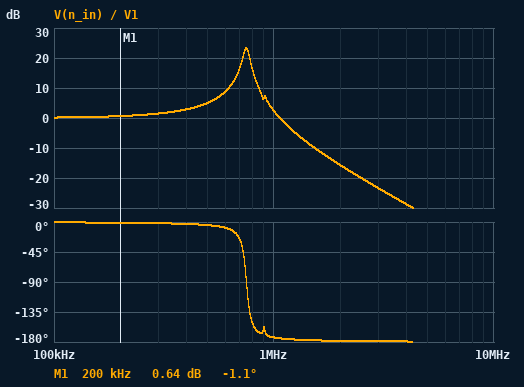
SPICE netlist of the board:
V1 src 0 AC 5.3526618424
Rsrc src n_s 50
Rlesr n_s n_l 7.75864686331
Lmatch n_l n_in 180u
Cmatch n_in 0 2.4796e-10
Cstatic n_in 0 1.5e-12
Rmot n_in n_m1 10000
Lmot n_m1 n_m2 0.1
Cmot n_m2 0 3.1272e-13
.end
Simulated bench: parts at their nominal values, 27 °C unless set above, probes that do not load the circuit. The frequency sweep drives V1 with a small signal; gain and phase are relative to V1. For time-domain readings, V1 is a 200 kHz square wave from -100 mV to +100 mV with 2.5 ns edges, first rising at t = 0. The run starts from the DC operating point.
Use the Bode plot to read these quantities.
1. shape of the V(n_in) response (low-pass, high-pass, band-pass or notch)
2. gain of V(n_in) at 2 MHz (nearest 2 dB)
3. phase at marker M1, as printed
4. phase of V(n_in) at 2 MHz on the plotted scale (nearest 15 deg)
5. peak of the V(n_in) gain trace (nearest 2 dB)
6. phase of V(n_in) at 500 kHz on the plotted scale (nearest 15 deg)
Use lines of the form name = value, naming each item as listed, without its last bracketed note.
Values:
shape of the V(n_in) response = low-pass
gain of V(n_in) at 2 MHz = -16 dB
phase at marker M1, as printed = -1.1 deg
phase of V(n_in) at 2 MHz on the plotted scale = -180 deg
peak of the V(n_in) gain trace = 24 dB
phase of V(n_in) at 500 kHz on the plotted scale = 0 deg
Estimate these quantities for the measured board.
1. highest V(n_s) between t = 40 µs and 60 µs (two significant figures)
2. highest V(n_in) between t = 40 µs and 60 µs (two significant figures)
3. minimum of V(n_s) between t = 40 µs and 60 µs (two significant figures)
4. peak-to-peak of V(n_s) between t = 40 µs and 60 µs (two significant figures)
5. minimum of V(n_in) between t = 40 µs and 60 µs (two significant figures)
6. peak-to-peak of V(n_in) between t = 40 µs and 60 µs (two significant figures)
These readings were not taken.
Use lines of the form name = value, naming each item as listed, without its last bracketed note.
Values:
highest V(n_s) between t = 40 µs and 60 µs = 110 mV
highest V(n_in) between t = 40 µs and 60 µs = 220 mV
minimum of V(n_s) between t = 40 µs and 60 µs = -110 mV
peak-to-peak of V(n_s) between t = 40 µs and 60 µs = 210 mV
minimum of V(n_in) between t = 40 µs and 60 µs = -220 mV
peak-to-peak of V(n_in) between t = 40 µs and 60 µs = 440 mV
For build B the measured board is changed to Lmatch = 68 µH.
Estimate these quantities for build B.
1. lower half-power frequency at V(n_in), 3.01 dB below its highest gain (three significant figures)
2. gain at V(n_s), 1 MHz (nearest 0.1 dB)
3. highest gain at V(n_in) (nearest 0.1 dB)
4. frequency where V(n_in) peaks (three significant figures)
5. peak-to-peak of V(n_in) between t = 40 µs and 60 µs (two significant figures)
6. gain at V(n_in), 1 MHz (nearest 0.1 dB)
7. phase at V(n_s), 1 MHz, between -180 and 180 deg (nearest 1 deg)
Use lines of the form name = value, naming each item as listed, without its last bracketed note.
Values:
lower half-power frequency at V(n_in), 3.01 dB below its highest gain = 1.15 MHz
gain at V(n_s), 1 MHz = -0.3 dB
highest gain at V(n_in) = 19.1 dB
frequency where V(n_in) peaks = 1.22 MHz
peak-to-peak of V(n_in) between t = 40 µs and 60 µs = 450 mV
gain at V(n_in), 1 MHz = 9.2 dB
phase at V(n_s), 1 MHz, between -180 and 180 deg = -13 deg
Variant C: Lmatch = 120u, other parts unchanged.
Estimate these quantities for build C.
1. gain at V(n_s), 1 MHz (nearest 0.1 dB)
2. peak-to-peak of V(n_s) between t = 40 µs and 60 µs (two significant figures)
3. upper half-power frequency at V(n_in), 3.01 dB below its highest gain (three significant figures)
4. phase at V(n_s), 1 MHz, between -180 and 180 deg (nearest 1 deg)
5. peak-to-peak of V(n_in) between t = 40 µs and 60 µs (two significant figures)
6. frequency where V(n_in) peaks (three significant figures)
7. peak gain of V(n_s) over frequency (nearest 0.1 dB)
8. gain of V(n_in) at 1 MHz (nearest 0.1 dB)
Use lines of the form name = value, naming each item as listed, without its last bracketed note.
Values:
gain at V(n_s), 1 MHz = -1.0 dB
peak-to-peak of V(n_s) between t = 40 µs and 60 µs = 220 mV
upper half-power frequency at V(n_in), 3.01 dB below its highest gain = 963 kHz
phase at V(n_s), 1 MHz, between -180 and 180 deg = 23 deg
peak-to-peak of V(n_in) between t = 40 µs and 60 µs = 550 mV
frequency where V(n_in) peaks = 930 kHz
peak gain of V(n_s) over frequency = 0 dB
gain of V(n_in) at 1 MHz = 14.1 dB
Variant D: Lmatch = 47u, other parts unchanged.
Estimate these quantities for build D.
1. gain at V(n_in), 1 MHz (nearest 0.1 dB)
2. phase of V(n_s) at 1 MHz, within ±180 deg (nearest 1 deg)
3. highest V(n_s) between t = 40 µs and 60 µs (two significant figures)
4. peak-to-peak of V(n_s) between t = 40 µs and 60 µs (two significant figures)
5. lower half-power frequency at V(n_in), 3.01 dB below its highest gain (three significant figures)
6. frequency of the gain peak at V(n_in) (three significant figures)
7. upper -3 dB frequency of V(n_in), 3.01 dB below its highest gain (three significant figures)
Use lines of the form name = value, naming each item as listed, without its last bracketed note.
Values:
gain at V(n_in), 1 MHz = 5.2 dB
phase of V(n_s) at 1 MHz, within ±180 deg = -8 deg
highest V(n_s) between t = 40 µs and 60 µs = 120 mV
peak-to-peak of V(n_s) between t = 40 µs and 60 µs = 240 mV
lower half-power frequency at V(n_in), 3.01 dB below its highest gain = 1.36 MHz
frequency of the gain peak at V(n_in) = 1.46 MHz
upper -3 dB frequency of V(n_in), 3.01 dB below its highest gain = 1.56 MHz
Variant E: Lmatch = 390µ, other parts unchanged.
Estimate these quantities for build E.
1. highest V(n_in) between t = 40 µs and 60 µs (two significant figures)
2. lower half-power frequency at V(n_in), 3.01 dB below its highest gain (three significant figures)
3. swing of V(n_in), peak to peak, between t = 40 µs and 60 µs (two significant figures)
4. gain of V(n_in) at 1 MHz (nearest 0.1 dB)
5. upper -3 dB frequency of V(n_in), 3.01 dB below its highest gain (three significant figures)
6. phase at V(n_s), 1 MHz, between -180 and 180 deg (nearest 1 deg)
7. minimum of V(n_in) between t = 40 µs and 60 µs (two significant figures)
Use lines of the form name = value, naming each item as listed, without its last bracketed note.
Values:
highest V(n_in) between t = 40 µs and 60 µs = 250 mV
lower half-power frequency at V(n_in), 3.01 dB below its highest gain = 498 kHz
swing of V(n_in), peak to peak, between t = 40 µs and 60 µs = 510 mV
gain of V(n_in) at 1 MHz = -9.0 dB
upper -3 dB frequency of V(n_in), 3.01 dB below its highest gain = 521 kHz
phase at V(n_s), 1 MHz, between -180 and 180 deg = 2 deg
minimum of V(n_in) between t = 40 µs and 60 µs = -260 mV
